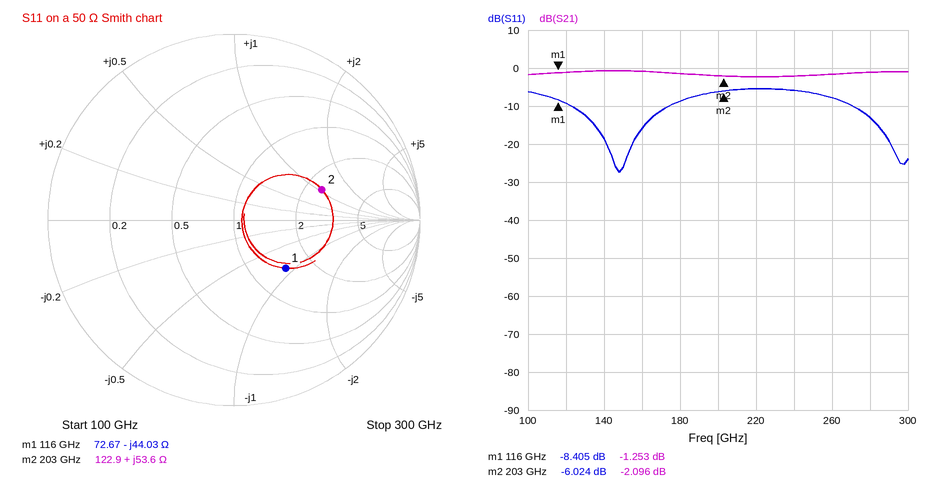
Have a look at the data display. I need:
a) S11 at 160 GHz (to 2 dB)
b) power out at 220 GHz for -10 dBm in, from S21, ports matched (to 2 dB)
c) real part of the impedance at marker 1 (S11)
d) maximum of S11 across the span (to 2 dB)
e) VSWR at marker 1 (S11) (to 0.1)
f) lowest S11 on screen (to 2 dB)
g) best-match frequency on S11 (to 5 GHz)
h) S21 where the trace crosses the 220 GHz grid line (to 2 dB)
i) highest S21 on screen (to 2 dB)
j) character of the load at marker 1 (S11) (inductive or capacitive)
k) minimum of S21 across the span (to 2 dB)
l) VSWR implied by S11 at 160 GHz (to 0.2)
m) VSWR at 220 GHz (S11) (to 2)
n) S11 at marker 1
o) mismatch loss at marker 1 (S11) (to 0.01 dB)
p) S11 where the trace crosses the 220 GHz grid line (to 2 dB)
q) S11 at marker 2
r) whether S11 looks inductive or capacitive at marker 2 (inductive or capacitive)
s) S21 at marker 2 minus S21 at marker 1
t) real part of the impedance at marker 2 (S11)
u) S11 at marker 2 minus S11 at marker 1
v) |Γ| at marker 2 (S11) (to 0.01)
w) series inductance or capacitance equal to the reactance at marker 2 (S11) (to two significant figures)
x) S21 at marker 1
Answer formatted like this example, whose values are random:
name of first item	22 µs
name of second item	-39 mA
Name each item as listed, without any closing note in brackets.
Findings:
S11 at 160 GHz	-16 dB
power out at 220 GHz for -10 dBm in, from S21, ports matched	-12 dBm
real part of the impedance at marker 1	72.67 Ω
maximum of S11 across the span	-6 dB
VSWR at marker 1 (S11)	2.2
lowest S11 on screen	-28 dB
best-match frequency on S11	150 GHz
S21 where the trace crosses the 220 GHz grid line	-2 dB
highest S21 on screen	0 dB
character of the load at marker 1 (S11)	capacitive
minimum of S21 across the span	-2 dB
VSWR implied by S11 at 160 GHz	1.4
VSWR at 220 GHz (S11)	4
S11 at marker 1	-8.405 dB
mismatch loss at marker 1 (S11)	0.68 dB
S11 where the trace crosses the 220 GHz grid line	-6 dB
S11 at marker 2	-6.024 dB
whether S11 looks inductive or capacitive at marker 2	inductive
S21 at marker 2 minus S21 at marker 1	-0.843 dB
real part of the impedance at marker 2	122.9 Ω
S11 at marker 2 minus S11 at marker 1	2.381 dB
|Γ| at marker 2 (S11)	0.50
series inductance or capacitance equal to the reactance at marker 2 (S11)	42 pH
S21 at marker 1	-1.253 dB
